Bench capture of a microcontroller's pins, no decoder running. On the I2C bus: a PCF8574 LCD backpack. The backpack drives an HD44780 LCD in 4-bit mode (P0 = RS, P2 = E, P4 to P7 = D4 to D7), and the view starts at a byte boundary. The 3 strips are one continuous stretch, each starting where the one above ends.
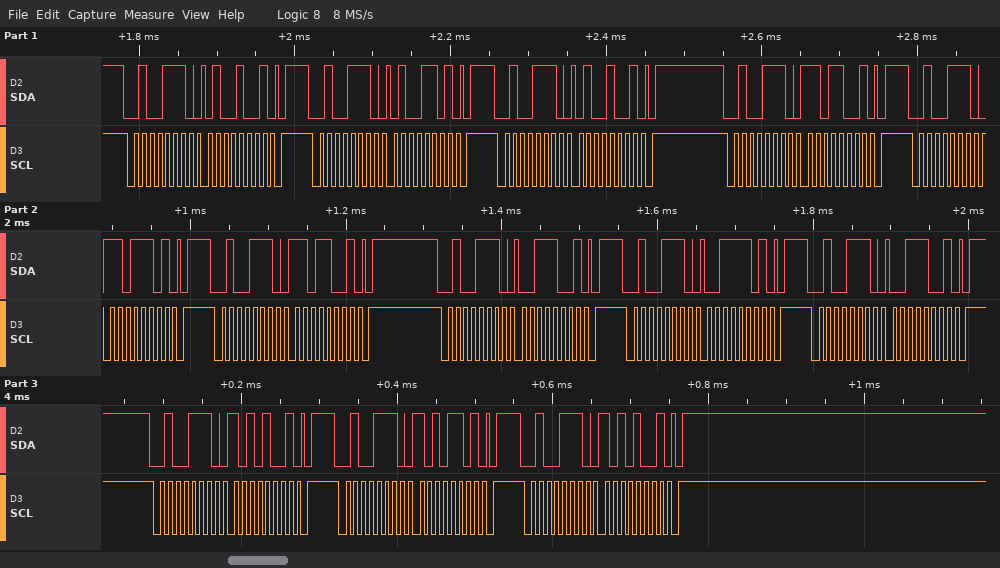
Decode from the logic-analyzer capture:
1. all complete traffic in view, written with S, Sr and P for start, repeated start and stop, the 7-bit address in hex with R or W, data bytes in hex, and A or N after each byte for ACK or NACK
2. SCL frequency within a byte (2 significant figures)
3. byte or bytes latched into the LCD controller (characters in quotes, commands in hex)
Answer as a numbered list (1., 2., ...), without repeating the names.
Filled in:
1. S 27W A 49 A P S 27W A 4D A P S 27W A 49 A P S 27W A D9 A P S 27W A DD A P S 27W A D9 A P S 27W A 39 A P S 27W A 3D A P S 27W A 39 A P S 27W A A9 A P S 27W A AD A P S 27W A A9 A P
2. 100 kHz
3. 'M' ':'
